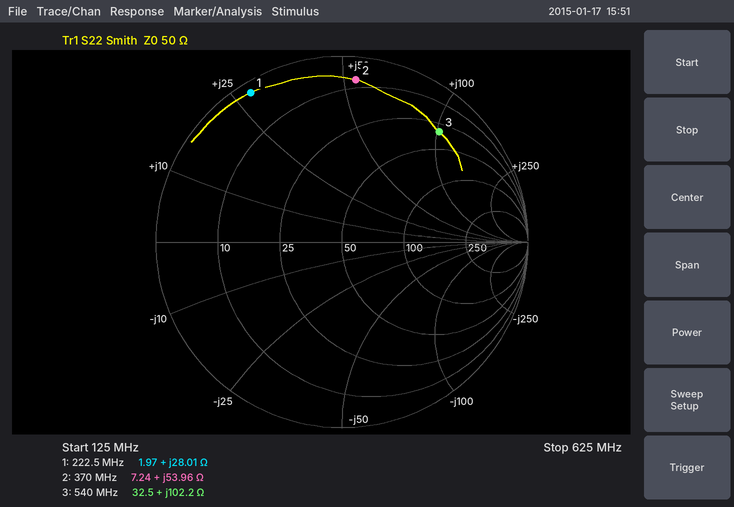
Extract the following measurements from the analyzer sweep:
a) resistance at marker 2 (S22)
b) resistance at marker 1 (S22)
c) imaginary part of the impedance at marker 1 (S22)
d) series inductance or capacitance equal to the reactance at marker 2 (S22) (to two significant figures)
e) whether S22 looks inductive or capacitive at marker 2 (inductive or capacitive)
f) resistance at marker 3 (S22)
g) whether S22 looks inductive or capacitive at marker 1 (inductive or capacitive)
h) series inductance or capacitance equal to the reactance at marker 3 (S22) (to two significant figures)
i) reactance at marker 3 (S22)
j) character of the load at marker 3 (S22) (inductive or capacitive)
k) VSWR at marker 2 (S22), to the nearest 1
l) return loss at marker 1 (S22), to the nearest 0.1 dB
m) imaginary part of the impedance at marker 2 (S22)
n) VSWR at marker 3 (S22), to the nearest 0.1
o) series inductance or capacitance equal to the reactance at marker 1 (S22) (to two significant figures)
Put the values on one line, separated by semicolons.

7.24 Ω; 1.97 Ω; +28.01 Ω; 23 nH; inductive; 32.5 Ω; inductive; 30 nH; +102.2 Ω; inductive; 15; 0.5 dB; +53.96 Ω; 8.5; 20 nH
